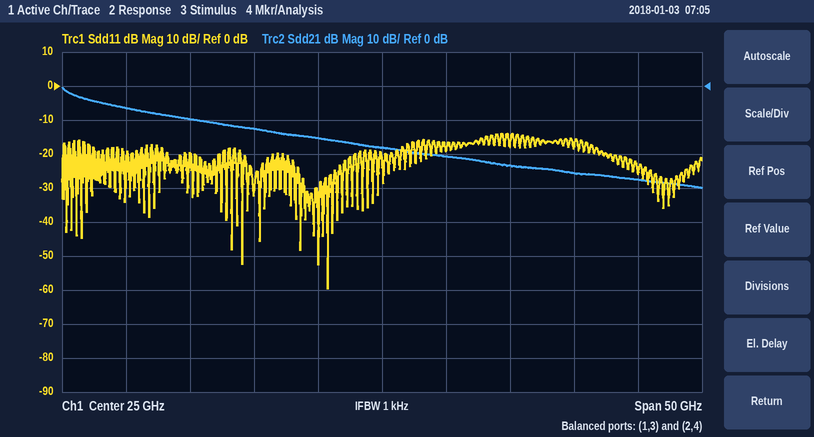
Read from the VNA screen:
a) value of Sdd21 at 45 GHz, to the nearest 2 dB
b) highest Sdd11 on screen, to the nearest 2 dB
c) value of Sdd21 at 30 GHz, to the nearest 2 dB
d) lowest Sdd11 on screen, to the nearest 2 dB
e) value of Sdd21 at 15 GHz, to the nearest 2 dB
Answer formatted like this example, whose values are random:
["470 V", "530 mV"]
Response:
["-28 dB", "-14 dB", "-20 dB", "-60 dB", "-12 dB"]
